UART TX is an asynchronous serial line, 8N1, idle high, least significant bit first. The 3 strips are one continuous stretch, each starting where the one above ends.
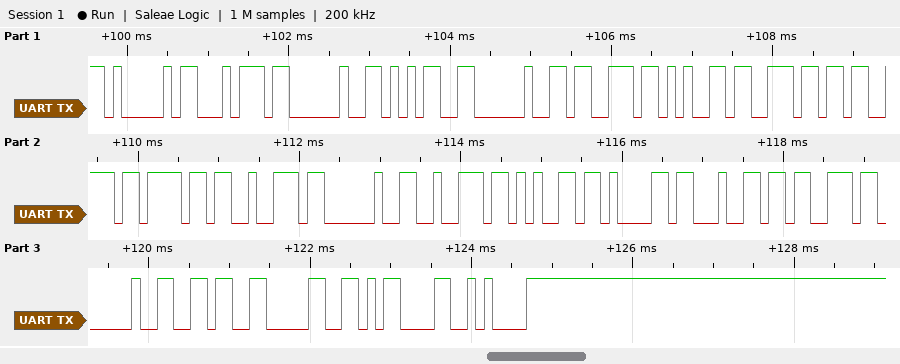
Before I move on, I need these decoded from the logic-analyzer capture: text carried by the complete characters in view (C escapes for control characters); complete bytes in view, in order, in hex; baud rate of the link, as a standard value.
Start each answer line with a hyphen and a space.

- "At 5 sensor reads 60\r\n"
- 41 74 20 35 20 73 65 6E 73 6F 72 20 72 65 61 64 73 20 36 30 0D 0A
- 9600 baud
